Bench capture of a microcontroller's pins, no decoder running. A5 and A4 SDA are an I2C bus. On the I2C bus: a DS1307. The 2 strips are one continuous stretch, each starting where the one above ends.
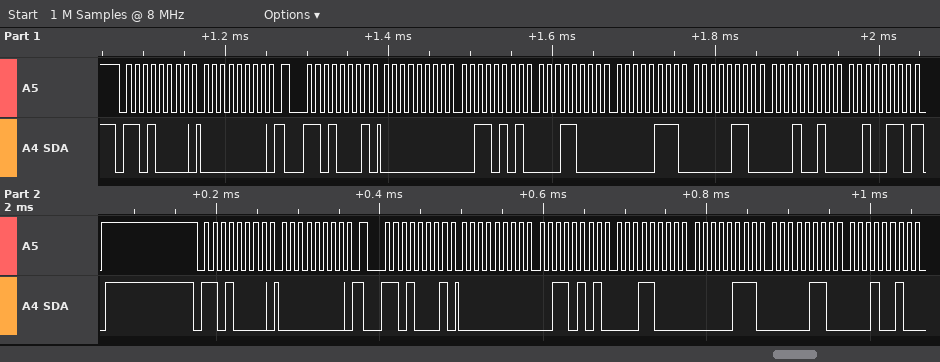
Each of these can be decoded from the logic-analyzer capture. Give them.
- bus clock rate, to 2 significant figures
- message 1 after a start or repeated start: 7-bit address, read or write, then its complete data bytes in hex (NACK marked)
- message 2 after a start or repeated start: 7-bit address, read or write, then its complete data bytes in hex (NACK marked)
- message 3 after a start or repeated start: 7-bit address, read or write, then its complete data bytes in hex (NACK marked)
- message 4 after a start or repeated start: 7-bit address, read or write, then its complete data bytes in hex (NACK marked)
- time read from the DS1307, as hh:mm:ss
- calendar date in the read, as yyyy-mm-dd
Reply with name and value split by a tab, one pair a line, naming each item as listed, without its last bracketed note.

bus clock rate, to 2 significant figures	100 kHz
message 1 after a start or repeated start: 7-bit address, read or write, then its complete data bytes in hex	0x68 write: 00
message 2 after a start or repeated start: 7-bit address, read or write, then its complete data bytes in hex	0x68 read: 00 35 18 07 06 12 26 NACK
message 3 after a start or repeated start: 7-bit address, read or write, then its complete data bytes in hex	0x68 write: 00
message 4 after a start or repeated start: 7-bit address, read or write, then its complete data bytes in hex	0x68 read: 00 35 18 07 06 12
time read from the DS1307, as hh:mm:ss	18:35:00
calendar date in the read, as yyyy-mm-dd	2026-12-06
